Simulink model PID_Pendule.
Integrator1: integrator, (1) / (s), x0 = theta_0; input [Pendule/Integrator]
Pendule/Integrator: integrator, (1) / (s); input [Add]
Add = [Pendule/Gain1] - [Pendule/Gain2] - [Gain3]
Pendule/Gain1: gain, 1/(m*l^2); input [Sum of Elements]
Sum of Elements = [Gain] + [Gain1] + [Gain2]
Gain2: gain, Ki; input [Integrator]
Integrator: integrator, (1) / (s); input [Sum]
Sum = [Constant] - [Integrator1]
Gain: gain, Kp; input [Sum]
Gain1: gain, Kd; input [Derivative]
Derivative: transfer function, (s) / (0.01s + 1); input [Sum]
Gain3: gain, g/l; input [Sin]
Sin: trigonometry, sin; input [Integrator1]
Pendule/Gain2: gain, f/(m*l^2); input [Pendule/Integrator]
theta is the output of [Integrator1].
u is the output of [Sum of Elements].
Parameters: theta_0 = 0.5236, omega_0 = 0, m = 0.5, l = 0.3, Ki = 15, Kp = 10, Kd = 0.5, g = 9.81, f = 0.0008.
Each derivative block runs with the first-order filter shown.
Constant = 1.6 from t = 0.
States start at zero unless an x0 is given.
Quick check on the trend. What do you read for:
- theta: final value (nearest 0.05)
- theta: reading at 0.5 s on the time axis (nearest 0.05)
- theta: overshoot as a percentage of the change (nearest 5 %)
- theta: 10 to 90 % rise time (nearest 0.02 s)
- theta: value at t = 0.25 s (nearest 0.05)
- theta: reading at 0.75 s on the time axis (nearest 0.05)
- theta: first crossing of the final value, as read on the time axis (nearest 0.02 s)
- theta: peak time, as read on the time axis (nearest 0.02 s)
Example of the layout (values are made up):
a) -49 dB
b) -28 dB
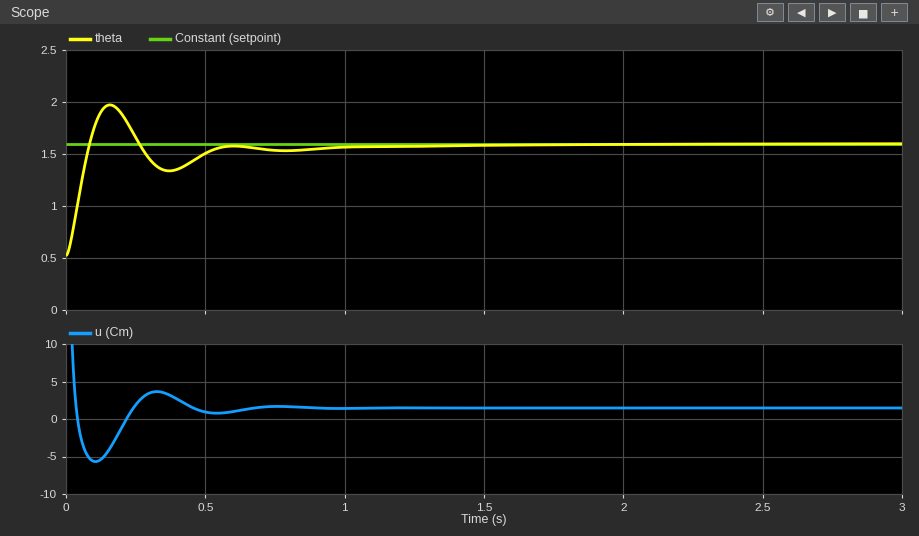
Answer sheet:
a) 1.60
b) 1.50
c) 35 %
d) 0.06 s
e) 1.65
f) 1.55
g) 0.08 s
h) 0.16 s
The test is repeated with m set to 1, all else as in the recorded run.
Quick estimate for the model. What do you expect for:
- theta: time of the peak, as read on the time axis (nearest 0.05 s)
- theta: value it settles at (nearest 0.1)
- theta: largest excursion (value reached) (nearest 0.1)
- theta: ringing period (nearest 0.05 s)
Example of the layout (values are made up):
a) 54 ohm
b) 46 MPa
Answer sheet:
a) 0.25 s
b) 1.6
c) 1.9
d) 0.60 s
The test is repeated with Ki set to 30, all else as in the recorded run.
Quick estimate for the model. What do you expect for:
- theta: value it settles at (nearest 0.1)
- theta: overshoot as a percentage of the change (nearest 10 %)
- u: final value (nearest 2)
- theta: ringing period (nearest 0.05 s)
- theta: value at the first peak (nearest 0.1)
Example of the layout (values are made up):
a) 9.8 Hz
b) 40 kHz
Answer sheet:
a) 1.6
b) 40 %
c) 2
d) 0.45 s
e) 2.0
